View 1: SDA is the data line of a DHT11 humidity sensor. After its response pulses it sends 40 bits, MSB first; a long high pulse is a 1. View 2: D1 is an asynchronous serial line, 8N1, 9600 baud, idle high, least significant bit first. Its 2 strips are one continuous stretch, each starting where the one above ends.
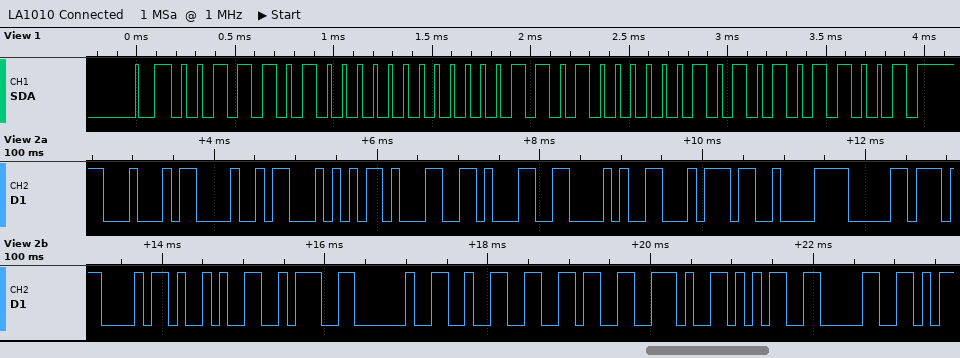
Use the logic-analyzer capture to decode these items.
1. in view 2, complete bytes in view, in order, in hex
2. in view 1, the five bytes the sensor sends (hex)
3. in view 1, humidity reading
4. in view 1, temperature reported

44 48 54 31 31 28 74 C2 B0 43 29 3A 20 32 36 2E 35 30
3A 00 1A 05 59
58 %
26.5 °C
